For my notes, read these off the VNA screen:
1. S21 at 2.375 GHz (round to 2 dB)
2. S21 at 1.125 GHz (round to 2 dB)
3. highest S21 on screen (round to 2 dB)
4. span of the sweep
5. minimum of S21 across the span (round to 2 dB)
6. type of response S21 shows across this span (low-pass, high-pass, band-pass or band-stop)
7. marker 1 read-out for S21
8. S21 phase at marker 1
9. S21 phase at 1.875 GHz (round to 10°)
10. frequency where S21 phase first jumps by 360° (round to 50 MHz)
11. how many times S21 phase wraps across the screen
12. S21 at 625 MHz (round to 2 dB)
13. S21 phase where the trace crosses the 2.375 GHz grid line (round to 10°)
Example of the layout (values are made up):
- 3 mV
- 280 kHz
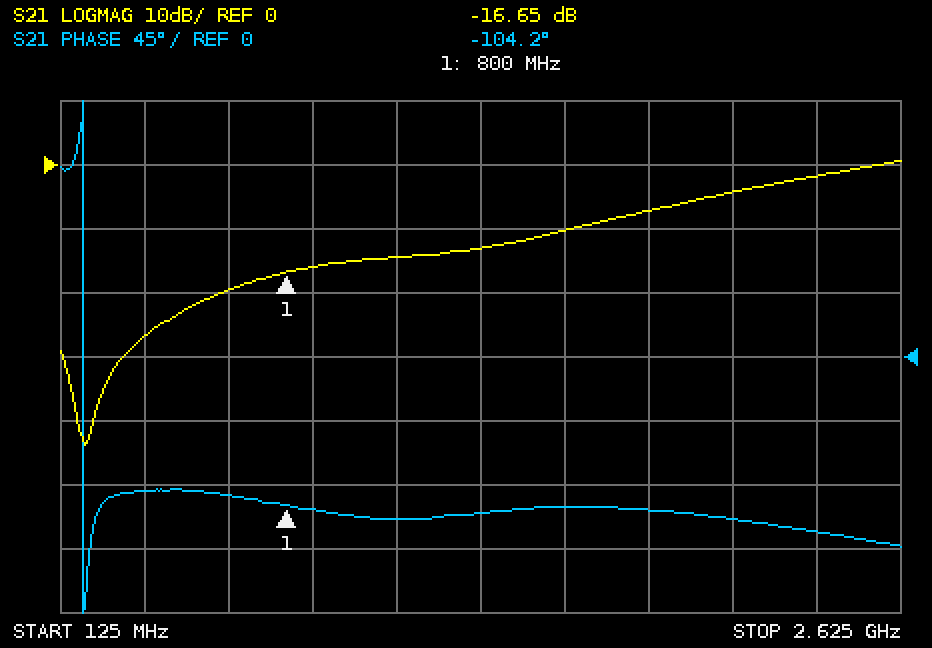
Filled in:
- -2 dB
- -14 dB
- 0 dB
- 2.5 GHz
- -44 dB
- high-pass
- -16.65 dB
- -104.2°
- -110°
- 200 MHz
- 1
- -20 dB
- -120°
